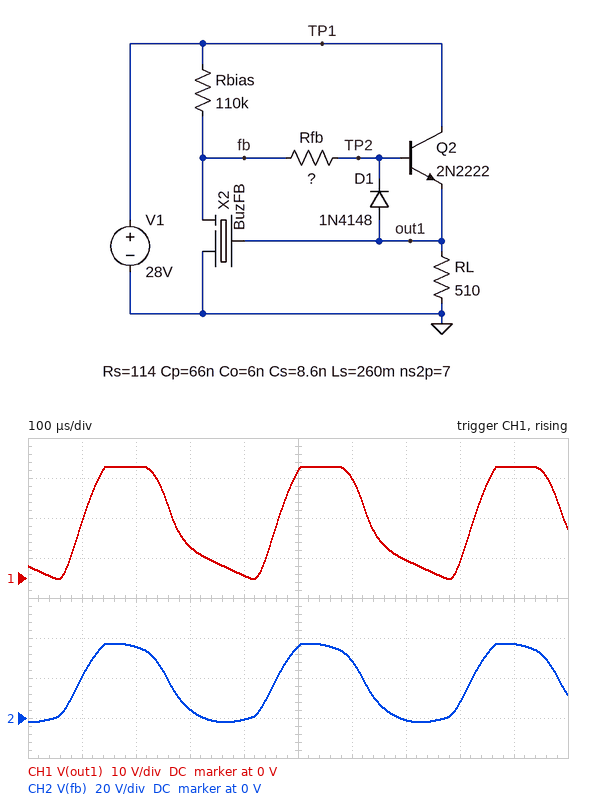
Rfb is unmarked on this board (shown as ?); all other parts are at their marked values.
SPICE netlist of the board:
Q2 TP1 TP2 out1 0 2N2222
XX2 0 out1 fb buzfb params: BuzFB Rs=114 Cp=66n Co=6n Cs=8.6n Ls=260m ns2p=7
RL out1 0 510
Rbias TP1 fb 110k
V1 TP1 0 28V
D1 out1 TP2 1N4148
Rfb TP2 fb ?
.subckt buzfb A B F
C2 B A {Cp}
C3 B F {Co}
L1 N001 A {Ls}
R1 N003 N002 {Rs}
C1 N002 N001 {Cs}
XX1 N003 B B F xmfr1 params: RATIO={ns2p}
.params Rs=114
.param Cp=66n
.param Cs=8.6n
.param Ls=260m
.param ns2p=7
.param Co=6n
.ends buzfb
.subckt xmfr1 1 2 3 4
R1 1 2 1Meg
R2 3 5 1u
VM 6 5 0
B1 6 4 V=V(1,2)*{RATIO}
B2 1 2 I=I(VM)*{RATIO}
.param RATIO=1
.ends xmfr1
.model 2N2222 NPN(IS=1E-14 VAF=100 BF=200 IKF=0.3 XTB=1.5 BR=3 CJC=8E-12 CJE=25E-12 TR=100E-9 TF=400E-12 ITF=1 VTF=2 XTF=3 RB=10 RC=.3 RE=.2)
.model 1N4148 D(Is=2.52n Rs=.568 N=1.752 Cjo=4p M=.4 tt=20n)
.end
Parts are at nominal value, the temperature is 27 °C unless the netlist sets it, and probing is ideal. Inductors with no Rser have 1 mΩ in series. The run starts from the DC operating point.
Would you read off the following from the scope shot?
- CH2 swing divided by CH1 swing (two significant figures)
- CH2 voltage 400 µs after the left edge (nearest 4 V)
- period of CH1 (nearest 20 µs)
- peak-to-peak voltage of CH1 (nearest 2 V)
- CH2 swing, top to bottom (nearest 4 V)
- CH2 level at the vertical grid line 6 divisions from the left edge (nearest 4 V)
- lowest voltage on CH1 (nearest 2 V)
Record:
1.4
0 V
360 µs
28 V
40 V
28 V
0 V
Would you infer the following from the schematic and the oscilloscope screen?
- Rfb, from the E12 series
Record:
18 kΩ
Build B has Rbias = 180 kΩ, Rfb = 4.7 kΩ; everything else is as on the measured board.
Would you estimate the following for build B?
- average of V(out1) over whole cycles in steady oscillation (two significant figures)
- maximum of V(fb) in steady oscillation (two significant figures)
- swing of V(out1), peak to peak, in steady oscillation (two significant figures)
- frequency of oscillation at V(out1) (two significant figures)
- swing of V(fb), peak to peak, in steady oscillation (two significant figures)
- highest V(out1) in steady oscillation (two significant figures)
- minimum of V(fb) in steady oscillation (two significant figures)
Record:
19 V
43 V
27 V
3.3 kHz
45 V
28 V
-1.7 V
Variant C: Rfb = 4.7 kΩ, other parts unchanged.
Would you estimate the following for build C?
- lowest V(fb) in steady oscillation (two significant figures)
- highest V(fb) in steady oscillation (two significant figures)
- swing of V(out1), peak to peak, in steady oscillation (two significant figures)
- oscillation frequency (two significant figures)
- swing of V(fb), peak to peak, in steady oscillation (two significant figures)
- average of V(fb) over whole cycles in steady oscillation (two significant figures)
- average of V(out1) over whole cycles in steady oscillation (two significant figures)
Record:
-1.3 V
43 V
27 V
3.3 kHz
45 V
20 V
19 V
